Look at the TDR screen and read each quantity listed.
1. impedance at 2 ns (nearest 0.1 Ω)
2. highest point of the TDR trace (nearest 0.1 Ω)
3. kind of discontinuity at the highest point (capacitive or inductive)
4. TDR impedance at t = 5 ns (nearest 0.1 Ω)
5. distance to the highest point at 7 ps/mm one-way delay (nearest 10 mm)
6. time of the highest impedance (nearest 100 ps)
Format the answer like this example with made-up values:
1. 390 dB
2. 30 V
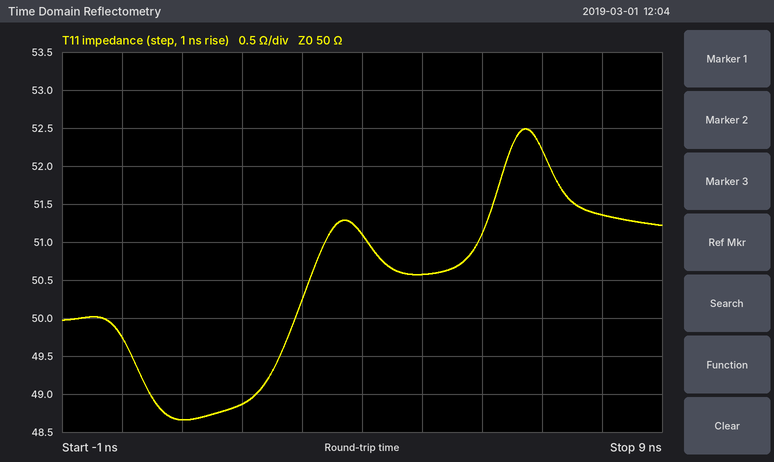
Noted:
1. 48.9 Ω
2. 52.5 Ω
3. inductive
4. 50.6 Ω
5. 480 mm
6. 6.7 ns
